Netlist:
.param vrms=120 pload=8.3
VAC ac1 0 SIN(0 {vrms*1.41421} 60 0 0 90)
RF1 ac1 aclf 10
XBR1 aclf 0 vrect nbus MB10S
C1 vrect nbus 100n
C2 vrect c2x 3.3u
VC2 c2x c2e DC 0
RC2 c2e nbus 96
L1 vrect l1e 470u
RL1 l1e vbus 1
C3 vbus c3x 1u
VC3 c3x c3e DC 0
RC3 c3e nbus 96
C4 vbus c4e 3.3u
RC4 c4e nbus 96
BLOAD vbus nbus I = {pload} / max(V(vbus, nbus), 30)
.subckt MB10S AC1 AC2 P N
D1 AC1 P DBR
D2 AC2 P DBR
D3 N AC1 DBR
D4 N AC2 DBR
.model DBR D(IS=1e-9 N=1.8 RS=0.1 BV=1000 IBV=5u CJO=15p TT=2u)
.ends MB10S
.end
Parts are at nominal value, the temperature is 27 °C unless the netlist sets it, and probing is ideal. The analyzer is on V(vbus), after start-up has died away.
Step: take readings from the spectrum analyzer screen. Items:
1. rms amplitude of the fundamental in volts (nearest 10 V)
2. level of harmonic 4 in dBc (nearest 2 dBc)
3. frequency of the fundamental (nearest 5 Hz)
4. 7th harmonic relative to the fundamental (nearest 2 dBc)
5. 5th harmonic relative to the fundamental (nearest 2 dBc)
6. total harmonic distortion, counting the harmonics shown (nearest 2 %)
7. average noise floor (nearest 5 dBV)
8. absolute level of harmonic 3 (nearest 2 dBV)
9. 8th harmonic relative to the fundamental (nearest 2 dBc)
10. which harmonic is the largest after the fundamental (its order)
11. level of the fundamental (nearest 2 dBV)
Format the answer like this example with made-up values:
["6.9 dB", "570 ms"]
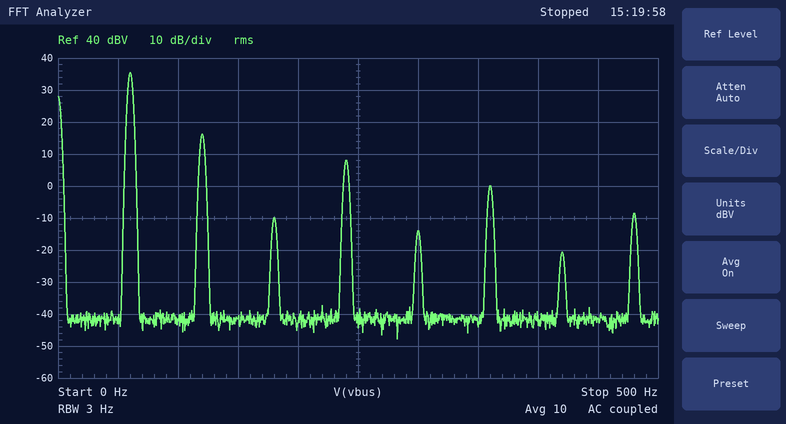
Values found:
["60 V", "-28 dBc", "60 Hz", "-56 dBc", "-50 dBc", "12 %", "-40 dBV", "-10 dBV", "-44 dBc", "2", "36 dBV"]
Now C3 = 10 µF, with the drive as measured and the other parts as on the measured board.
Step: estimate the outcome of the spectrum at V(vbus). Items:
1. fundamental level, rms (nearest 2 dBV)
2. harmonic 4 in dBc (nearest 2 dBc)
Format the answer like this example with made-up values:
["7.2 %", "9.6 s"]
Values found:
["36 dBV", "-32 dBc"]
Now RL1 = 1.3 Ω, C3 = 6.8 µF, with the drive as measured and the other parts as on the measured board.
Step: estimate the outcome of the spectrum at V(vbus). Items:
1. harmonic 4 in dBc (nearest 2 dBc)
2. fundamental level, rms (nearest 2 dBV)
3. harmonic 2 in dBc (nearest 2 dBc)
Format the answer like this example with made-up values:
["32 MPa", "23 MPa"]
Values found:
["-30 dBc", "36 dBV", "-24 dBc"]
